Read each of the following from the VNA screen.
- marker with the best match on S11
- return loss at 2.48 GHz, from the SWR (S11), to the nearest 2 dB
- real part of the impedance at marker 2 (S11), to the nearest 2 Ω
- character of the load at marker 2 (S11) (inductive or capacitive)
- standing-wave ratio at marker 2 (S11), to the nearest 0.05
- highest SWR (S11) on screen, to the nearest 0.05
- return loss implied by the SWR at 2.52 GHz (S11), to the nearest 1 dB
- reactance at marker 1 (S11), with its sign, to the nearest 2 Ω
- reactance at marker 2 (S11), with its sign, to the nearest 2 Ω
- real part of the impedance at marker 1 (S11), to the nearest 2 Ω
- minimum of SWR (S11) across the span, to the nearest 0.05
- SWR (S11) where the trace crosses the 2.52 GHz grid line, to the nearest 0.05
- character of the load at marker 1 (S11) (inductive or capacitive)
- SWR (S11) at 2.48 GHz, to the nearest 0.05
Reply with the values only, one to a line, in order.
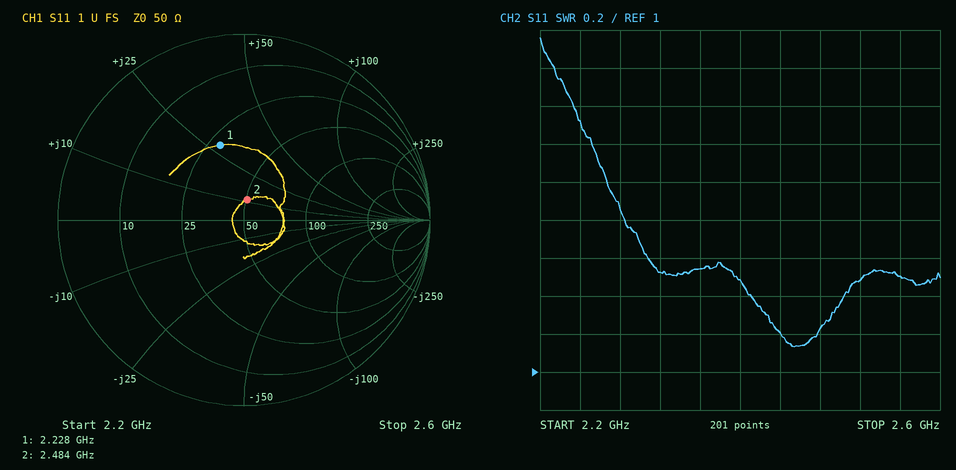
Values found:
marker 2
20 dB
50 Ω
inductive
1.25
2.75
14 dB
+28 Ω
+12 Ω
28 Ω
1.15
1.50
inductive
1.25
